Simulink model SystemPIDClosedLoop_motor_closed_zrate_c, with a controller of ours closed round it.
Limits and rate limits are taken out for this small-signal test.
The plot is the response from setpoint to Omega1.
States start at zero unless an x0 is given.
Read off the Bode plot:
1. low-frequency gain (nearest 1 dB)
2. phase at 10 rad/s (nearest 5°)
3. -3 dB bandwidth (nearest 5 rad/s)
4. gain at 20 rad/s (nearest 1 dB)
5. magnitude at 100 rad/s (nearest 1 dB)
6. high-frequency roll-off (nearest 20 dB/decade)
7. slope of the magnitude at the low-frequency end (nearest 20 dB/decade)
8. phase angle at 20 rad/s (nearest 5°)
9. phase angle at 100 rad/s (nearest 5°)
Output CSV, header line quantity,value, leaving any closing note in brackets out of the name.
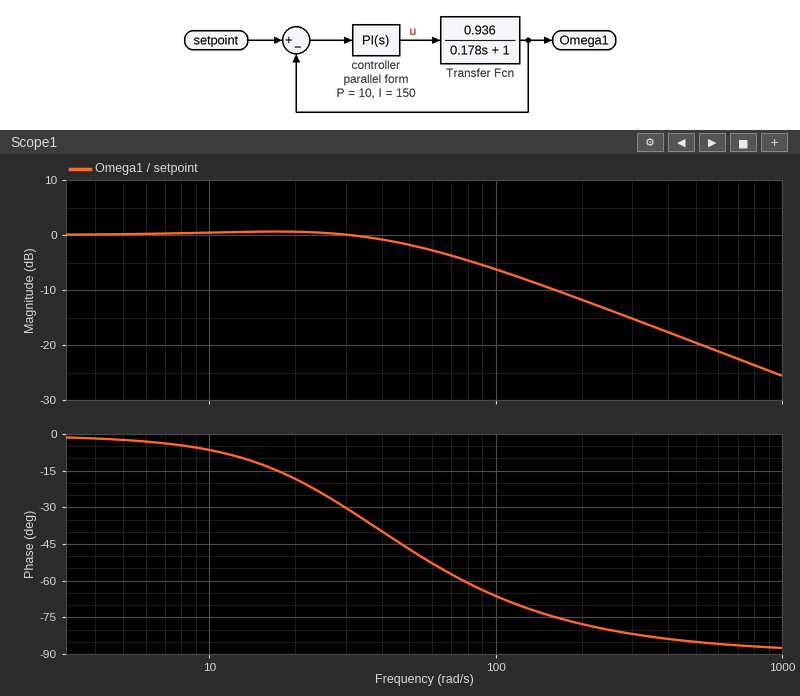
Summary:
quantity,value
low-frequency gain,0 dB
phase at 10 rad/s,-5°
-3 dB bandwidth,60 rad/s
gain at 20 rad/s,1 dB
magnitude at 100 rad/s,-6 dB
high-frequency roll-off,-20 dB/decade
slope of the magnitude at the low-frequency end,0 dB/decade
phase angle at 20 rad/s,-20°
phase angle at 100 rad/s,-65°
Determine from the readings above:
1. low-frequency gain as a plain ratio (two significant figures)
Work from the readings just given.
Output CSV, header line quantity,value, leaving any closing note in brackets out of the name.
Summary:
quantity,value
low-frequency gain as a plain ratio,1.0
